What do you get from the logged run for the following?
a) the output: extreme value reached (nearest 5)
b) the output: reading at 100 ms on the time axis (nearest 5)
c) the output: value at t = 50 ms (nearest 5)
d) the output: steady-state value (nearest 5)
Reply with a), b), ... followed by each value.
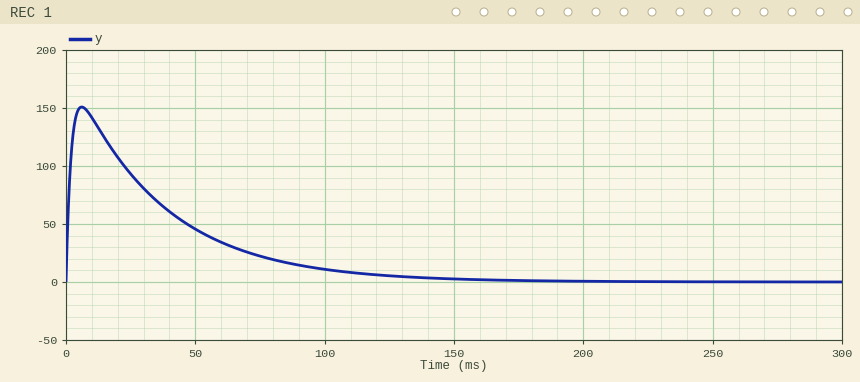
a) 150
b) 10
c) 45
d) 0
